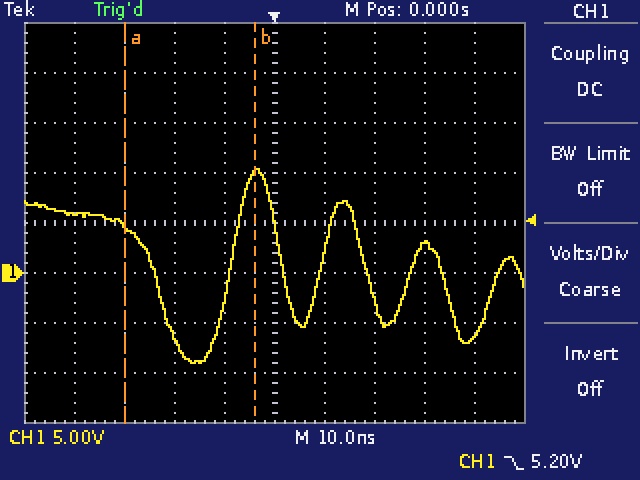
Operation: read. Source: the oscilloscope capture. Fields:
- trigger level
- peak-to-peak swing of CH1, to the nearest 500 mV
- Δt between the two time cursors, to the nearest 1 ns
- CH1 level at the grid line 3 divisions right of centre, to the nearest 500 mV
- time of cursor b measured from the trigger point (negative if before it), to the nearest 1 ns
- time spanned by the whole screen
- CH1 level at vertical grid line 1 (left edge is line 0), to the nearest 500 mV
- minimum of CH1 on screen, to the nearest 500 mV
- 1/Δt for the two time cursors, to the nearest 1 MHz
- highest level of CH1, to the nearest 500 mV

5.20 V
19.5 V
26 ns
3.0 V
-4 ns
100 ns
6.0 V
-9.0 V
38 MHz
10.5 V
